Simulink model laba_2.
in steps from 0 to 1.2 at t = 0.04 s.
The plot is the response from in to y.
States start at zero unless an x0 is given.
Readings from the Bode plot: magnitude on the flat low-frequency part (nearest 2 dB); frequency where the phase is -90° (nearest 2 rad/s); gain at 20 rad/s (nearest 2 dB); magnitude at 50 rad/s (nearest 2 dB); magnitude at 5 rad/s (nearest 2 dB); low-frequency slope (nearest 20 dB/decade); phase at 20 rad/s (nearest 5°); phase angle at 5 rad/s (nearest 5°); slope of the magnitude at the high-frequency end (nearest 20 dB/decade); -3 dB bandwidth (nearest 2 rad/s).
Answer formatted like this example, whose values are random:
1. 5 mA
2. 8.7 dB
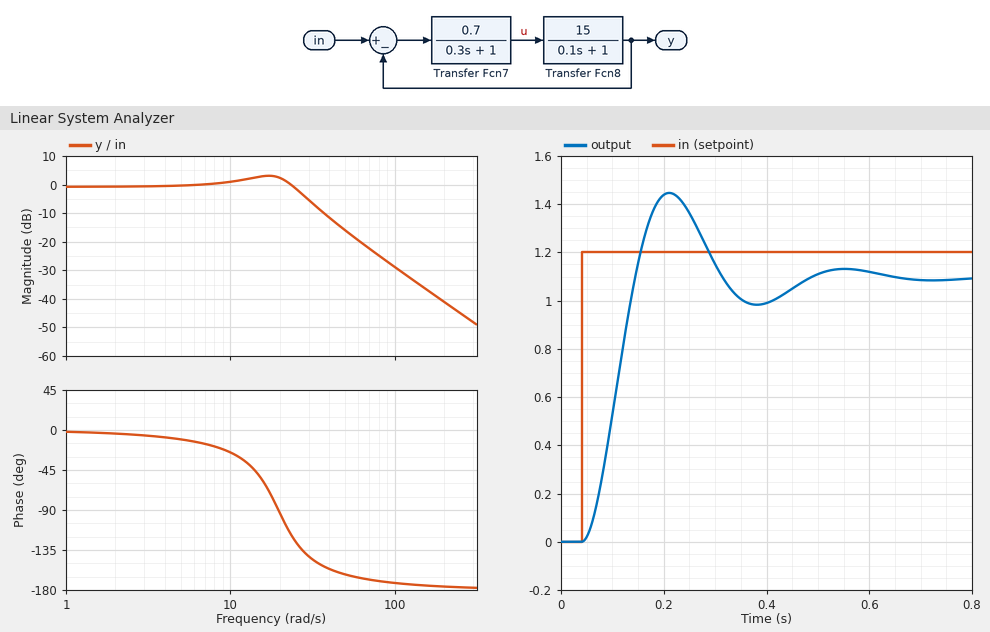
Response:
1. 0 dB
2. 20 rad/s
3. 2 dB
4. -16 dB
5. 0 dB
6. 0 dB/decade
7. -95°
8. -10°
9. -40 dB/decade
10. 28 rad/s
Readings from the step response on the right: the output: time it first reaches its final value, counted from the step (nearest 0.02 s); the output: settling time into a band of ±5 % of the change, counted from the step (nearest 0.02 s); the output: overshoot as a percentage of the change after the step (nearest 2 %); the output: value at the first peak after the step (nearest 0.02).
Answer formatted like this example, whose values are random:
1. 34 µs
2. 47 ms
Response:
1. 0.10 s
2. 0.40 s
3. 32 %
4. 1.44
